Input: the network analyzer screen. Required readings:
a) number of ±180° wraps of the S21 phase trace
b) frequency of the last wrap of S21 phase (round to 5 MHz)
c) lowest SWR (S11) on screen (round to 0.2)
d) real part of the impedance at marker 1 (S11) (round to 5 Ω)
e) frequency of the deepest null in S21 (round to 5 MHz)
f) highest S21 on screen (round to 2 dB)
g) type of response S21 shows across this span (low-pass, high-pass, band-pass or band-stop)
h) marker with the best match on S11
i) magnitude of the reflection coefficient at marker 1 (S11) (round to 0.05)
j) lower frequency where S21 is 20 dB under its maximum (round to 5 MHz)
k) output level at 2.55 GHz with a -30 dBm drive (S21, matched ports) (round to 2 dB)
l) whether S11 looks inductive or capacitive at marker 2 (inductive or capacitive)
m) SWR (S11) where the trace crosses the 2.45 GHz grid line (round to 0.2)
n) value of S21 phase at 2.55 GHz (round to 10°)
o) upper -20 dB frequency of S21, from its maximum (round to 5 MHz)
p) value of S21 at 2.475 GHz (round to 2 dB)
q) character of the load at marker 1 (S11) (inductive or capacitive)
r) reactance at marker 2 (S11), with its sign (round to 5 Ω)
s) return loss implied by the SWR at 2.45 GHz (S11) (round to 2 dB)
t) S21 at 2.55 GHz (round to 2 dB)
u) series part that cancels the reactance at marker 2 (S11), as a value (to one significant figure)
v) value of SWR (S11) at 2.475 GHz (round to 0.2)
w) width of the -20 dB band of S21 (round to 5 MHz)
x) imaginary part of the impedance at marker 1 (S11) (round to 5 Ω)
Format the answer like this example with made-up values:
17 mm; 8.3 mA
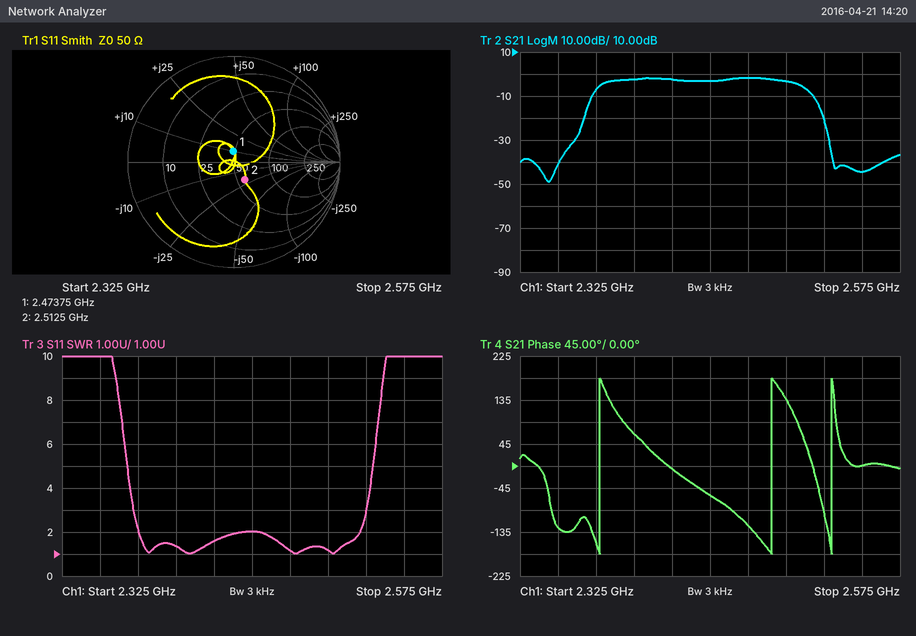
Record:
3; 2.530 GHz; 1.0; 50 Ω; 2.345 GHz; -2 dB; band-pass; marker 1; 0.10; 2.365 GHz; -74 dBm; capacitive; 2.0; 0°; 2.525 GHz; -2 dB; inductive; -20 Ω; 10 dB; -44 dB; 1 nH; 1.2; 160 MHz; +10 Ω
